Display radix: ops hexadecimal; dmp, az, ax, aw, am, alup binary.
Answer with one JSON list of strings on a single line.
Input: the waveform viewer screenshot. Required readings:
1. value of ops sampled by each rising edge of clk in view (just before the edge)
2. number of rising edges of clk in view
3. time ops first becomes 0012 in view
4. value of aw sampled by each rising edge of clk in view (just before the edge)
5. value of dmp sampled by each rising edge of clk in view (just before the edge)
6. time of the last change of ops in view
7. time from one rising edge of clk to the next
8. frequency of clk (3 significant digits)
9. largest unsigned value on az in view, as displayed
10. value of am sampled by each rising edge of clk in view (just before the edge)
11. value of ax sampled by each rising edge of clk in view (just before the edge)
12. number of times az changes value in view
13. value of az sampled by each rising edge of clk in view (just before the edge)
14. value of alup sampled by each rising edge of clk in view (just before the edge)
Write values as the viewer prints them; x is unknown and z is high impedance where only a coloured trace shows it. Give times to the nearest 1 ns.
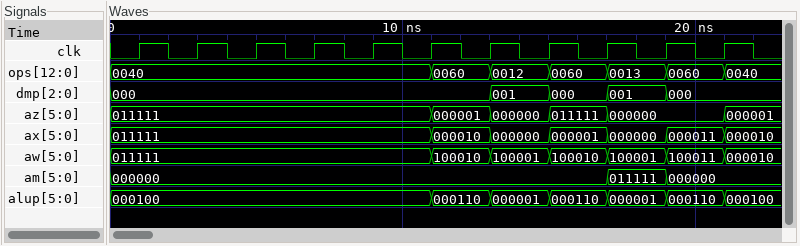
["0040, 0040, 0040, 0040, 0040, 0040, 0060, 0012, 0060, 0013, 0060", "11", "13 ns", "011111, 011111, 011111, 011111, 011111, 011111, 100010, 100001, 100010, 100001, 100011", "000, 000, 000, 000, 000, 000, 000, 001, 000, 001, 000", "21 ns", "2 ns", "500 MHz", "011111", "000000, 000000, 000000, 000000, 000000, 000000, 000000, 000000, 000000, 011111, 000000", "011111, 011111, 011111, 011111, 011111, 011111, 000010, 000000, 000001, 000000, 000011", "5", "011111, 011111, 011111, 011111, 011111, 011111, 000001, 000000, 011111, 000000, 000000", "000100, 000100, 000100, 000100, 000100, 000100, 000110, 000001, 000110, 000001, 000110"]
